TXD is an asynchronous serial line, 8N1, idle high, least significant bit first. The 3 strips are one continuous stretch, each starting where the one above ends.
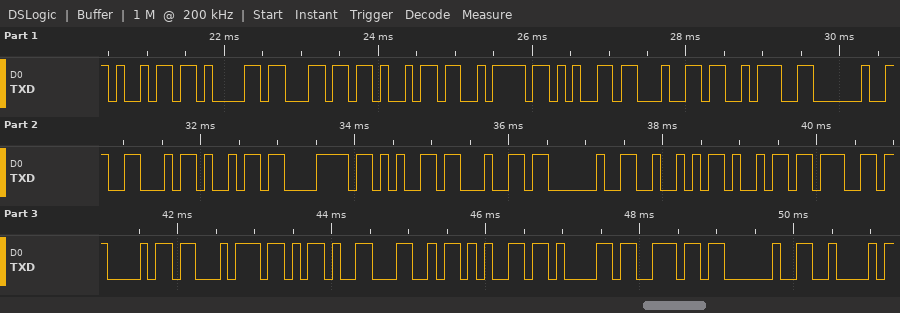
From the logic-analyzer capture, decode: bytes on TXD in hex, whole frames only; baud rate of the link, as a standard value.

0x69 0x61 0x6C 0x69 0x7A 0x65 0x64 0x3A 0x20 0x46 0x69 0x78 0x65 0x64 0x20 0x52 0x69 0x67 0x68 0x74 0x2D 0x4C 0x65 0x61 0x6E 0x20 0x42
9600 baud
